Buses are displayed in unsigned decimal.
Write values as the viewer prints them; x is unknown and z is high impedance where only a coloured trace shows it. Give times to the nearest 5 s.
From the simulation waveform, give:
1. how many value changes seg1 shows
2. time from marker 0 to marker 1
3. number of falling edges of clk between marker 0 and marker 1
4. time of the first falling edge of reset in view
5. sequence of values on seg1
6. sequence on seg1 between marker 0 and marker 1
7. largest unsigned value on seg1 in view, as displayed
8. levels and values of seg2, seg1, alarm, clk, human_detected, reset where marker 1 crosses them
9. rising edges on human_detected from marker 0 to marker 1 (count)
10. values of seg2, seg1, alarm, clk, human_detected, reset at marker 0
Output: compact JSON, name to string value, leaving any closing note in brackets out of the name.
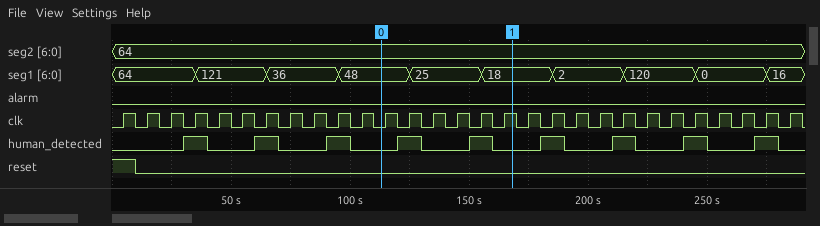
{"how many value changes seg1 shows": "9", "time from marker 0 to marker 1": "55 s", "number of falling edges of clk between marker 0 and marker 1": "5", "time of the first falling edge of reset in view": "10 s", "sequence of values on seg1": "64, 121, 36, 48, 25, 18, 2, 120, 0, 16", "sequence on seg1 between marker 0 and marker 1": "48, 25, 18", "largest unsigned value on seg1 in view, as displayed": "121", "levels and values of seg2, seg1, alarm, clk, human_detected, reset where marker 1 crosses them": "seg2=64, seg1=18, alarm=0, clk=1, human_detected=0, reset=0", "rising edges on human_detected from marker 0 to marker 1": "2", "values of seg2, seg1, alarm, clk, human_detected, reset at marker 0": "seg2=64, seg1=48, alarm=0, clk=0, human_detected=0, reset=0"}
